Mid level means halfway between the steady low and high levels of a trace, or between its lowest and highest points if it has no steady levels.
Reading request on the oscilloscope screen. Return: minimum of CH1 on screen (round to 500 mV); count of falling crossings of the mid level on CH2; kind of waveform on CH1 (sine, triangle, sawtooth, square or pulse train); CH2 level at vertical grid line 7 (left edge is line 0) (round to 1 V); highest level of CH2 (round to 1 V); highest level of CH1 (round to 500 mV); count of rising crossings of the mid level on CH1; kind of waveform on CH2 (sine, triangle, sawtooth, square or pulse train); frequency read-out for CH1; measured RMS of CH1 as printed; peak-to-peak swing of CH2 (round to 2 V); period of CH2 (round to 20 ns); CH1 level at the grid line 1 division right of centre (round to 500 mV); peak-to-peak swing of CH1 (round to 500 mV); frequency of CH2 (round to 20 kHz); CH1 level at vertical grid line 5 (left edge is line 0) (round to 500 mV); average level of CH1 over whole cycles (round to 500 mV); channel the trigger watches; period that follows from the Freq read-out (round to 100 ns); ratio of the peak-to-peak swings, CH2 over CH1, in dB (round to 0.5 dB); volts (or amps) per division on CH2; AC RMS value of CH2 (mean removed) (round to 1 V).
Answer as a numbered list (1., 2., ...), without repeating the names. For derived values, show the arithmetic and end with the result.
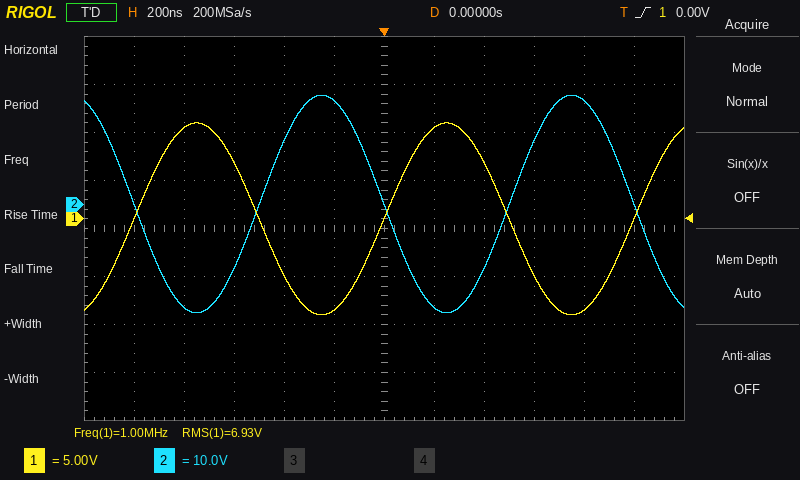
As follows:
1. -10.0 V
2. 3
3. sine
4. -21 V
5. 23 V
6. 10.0 V
7. 3
8. sine
9. 1.00 MHz
10. 6.93 V
11. 46 V
12. 1.00 µs
13. 9.5 V
14. 10.0 V − (-10.0 V) = 20.0 V
15. 1 / 1.00 µs ≈ 1.00 MHz
16. -9.5 V
17. (10.0 V + (-10.0 V)) / 2 ≈ 0.0 V
18. CH1
19. 1 / 1.00 MHz ≈ 1.0 µs
20. 20 log10(46 V / 20.0 V) ≈ 7.23 dB, so 7.0 dB to the nearest 0.5 dB
21. 10 V
22. 46 V / (2√2) ≈ 16 V
